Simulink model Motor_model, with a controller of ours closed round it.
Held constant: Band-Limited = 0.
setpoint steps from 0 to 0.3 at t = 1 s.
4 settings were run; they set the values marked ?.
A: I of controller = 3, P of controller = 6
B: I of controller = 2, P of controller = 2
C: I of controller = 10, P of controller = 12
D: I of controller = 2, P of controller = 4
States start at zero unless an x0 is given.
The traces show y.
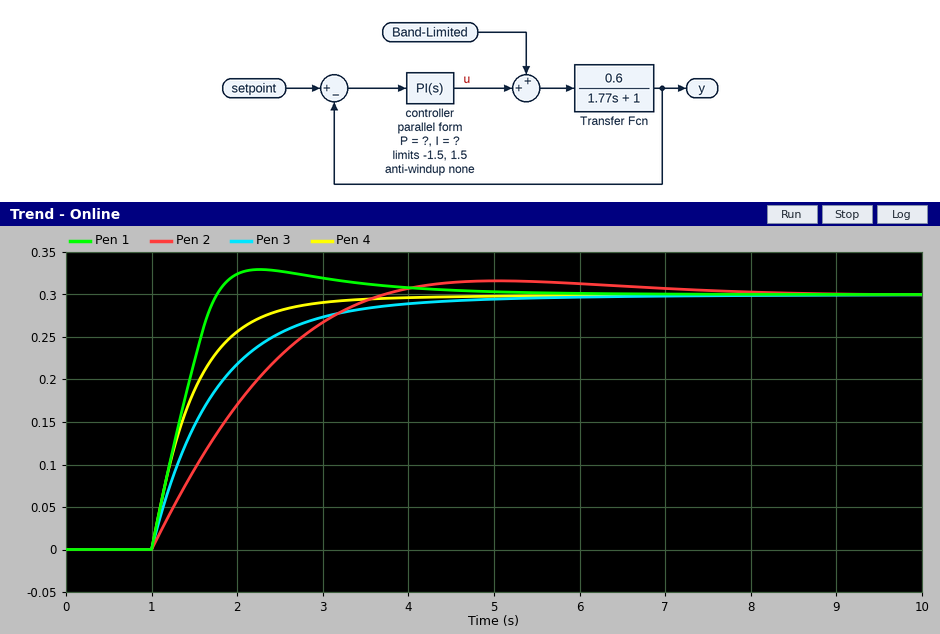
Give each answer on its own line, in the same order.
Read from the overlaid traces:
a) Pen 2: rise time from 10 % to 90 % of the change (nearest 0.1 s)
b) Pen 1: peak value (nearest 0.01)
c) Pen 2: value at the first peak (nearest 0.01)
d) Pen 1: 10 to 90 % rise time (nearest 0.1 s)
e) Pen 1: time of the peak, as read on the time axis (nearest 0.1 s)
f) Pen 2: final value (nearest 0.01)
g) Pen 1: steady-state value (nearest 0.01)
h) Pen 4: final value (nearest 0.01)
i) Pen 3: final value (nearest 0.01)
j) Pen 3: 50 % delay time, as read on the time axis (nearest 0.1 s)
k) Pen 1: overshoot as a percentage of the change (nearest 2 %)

1.9 s
0.33
0.32
0.6 s
2.3 s
0.30
0.30
0.30
0.30
1.5 s
10 %
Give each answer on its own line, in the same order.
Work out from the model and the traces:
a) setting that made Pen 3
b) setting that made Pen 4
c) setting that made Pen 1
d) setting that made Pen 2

D
A
C
B
